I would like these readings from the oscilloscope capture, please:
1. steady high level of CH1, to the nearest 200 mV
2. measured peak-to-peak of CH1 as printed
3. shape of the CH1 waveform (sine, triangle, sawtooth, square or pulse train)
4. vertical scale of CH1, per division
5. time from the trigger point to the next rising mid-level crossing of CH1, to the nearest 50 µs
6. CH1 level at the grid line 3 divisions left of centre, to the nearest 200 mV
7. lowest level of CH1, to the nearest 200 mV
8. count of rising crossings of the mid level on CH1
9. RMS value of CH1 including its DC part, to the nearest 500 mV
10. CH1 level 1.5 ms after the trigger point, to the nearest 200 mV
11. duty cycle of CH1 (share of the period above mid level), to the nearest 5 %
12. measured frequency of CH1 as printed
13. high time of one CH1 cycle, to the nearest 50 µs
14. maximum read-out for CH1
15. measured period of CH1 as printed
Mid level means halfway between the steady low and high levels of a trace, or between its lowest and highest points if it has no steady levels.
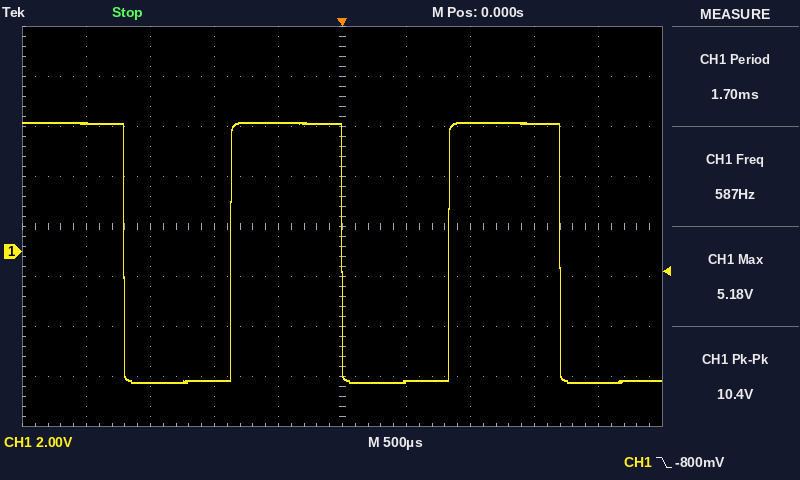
5.2 V
10.4 V
square
2 V
850 µs
-5.2 V
-5.2 V
2
5.0 V
5.2 V
50 %
587 Hz
850 µs
5.18 V
1.70 ms
